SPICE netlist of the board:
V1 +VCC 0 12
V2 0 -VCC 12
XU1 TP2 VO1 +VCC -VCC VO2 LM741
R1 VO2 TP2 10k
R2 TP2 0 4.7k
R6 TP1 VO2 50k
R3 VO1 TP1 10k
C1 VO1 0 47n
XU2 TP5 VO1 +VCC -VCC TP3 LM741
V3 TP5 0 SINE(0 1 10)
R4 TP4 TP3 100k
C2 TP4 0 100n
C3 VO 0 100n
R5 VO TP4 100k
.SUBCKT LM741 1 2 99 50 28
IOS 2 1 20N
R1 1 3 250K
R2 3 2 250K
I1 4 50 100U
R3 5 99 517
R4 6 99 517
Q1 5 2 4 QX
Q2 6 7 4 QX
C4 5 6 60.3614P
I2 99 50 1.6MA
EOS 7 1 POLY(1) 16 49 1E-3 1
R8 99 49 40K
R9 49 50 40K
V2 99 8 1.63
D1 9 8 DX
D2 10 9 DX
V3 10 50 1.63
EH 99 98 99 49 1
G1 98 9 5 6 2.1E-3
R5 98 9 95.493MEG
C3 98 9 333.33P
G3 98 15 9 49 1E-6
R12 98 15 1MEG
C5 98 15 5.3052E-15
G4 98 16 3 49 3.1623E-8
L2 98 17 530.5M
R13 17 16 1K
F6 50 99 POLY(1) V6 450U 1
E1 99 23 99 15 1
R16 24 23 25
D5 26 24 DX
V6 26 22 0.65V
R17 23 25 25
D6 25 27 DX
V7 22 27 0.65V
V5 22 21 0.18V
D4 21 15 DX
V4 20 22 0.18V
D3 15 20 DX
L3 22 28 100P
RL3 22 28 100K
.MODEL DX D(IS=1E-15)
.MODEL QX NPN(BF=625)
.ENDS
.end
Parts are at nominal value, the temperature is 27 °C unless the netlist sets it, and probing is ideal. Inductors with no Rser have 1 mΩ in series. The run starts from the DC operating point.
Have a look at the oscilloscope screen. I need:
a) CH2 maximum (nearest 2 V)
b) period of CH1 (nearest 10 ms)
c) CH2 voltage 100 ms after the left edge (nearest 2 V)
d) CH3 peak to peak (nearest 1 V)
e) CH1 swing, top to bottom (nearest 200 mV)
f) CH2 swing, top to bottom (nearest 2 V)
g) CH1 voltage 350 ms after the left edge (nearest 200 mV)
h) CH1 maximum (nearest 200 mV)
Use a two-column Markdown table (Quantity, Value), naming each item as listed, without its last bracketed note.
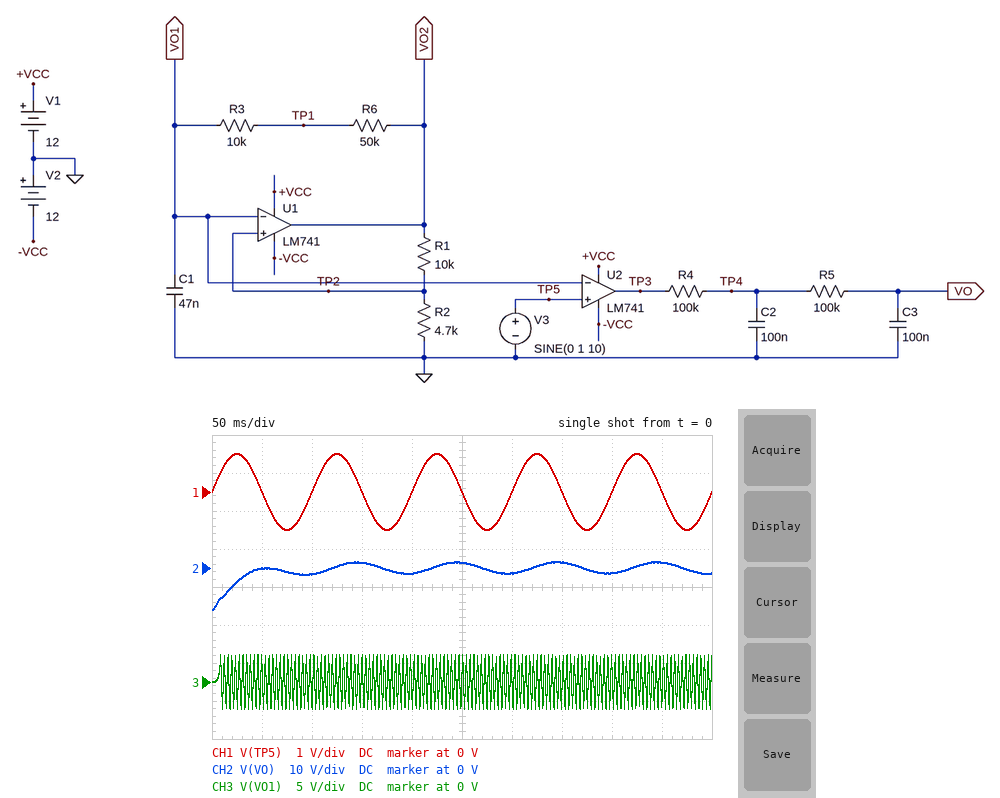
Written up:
| Quantity | Value |
|---|---|
| CH2 maximum | 2 V |
| period of CH1 | 100 ms |
| CH2 voltage 100 ms after the left edge | -2 V |
| CH3 peak to peak | 7 V |
| CH1 swing, top to bottom | 2.0 V |
| CH2 swing, top to bottom | 12 V |
| CH1 voltage 350 ms after the left edge | 0 V |
| CH1 maximum | 1.0 V |
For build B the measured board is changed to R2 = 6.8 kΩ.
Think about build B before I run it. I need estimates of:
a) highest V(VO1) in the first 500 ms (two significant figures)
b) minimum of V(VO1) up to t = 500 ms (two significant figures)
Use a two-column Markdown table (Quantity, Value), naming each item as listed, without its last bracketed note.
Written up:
| Quantity | Value |
|---|---|
| highest V(VO1) in the first 500 ms | 4.4 V |
| minimum of V(VO1) up to t = 500 ms | -4.4 V |
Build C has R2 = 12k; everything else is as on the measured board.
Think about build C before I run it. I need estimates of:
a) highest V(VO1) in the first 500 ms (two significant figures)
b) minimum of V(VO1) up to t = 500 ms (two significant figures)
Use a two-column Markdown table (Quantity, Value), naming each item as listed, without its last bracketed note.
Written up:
| Quantity | Value |
|---|---|
| highest V(VO1) in the first 500 ms | 6.0 V |
| minimum of V(VO1) up to t = 500 ms | -6.0 V |
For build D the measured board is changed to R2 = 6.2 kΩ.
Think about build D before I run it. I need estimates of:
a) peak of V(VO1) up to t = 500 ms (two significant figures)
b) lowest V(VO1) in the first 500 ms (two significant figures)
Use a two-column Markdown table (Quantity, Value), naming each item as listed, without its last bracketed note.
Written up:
| Quantity | Value |
|---|---|
| peak of V(VO1) up to t = 500 ms | 4.2 V |
| lowest V(VO1) in the first 500 ms | -4.2 V |
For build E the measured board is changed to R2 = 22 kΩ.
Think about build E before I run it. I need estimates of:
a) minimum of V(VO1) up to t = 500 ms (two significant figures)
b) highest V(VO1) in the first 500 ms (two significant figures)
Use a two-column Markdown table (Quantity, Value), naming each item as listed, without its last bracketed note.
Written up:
| Quantity | Value |
|---|---|
| minimum of V(VO1) up to t = 500 ms | -7.5 V |
| highest V(VO1) in the first 500 ms | 7.5 V |
